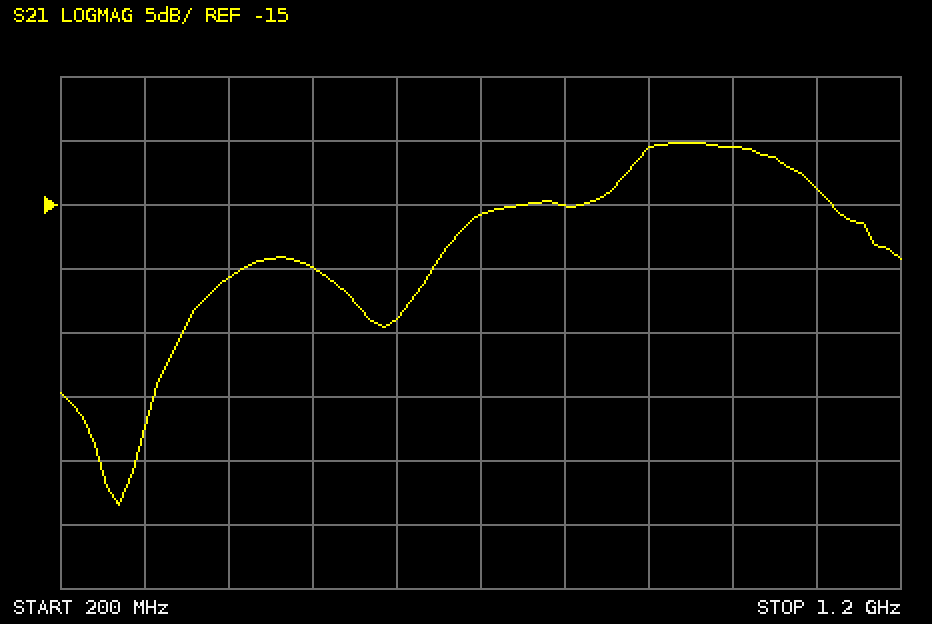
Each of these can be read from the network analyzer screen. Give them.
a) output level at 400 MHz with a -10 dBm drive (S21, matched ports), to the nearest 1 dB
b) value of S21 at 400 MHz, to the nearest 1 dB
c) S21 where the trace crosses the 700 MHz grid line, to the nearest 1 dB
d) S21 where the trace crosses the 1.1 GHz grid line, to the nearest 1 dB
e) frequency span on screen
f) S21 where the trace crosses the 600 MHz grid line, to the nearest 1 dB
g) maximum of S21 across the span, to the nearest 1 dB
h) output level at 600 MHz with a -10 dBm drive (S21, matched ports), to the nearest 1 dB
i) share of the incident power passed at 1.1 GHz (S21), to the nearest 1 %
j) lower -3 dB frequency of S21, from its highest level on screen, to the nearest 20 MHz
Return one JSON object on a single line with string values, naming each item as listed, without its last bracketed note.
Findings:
{"output level at 400 MHz with a -10 dBm drive (S21, matched ports), to the nearest 1 dB": "-31 dBm", "value of S21 at 400 MHz, to the nearest 1 dB": "-21 dB", "S21 where the trace crosses the 700 MHz grid line, to the nearest 1 dB": "-16 dB", "S21 where the trace crosses the 1.1 GHz grid line, to the nearest 1 dB": "-14 dB", "frequency span on screen": "1 GHz", "S21 where the trace crosses the 600 MHz grid line, to the nearest 1 dB": "-24 dB", "maximum of S21 across the span, to the nearest 1 dB": "-10 dB", "output level at 600 MHz with a -10 dBm drive (S21, matched ports), to the nearest 1 dB": "-34 dBm", "share of the incident power passed at 1.1 GHz (S21), to the nearest 1 %": "4 %", "lower -3 dB frequency of S21, from its highest level on screen, to the nearest 20 MHz": "860 MHz"}
